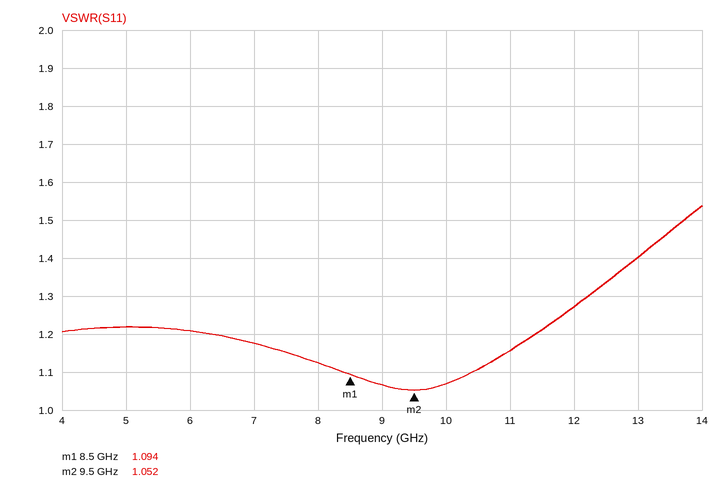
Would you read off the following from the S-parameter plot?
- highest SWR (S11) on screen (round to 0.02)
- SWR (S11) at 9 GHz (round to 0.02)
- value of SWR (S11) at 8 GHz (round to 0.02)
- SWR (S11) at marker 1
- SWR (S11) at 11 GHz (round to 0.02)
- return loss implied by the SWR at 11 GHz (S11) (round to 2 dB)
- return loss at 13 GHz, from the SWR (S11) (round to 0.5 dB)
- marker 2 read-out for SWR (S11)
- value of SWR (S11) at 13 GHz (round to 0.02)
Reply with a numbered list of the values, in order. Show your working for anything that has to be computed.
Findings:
1. 1.54
2. 1.06
3. 1.12
4. 1.094
5. 1.16
6. −20 log10((1.16 − 1)/(1.16 + 1)) ≈ 22.6 dB, so 22 dB to the nearest 2 dB
7. −20 log10((1.4 − 1)/(1.4 + 1)) ≈ 15.6 dB, so 15.5 dB to the nearest 0.5 dB
8. 1.052
9. 1.40
